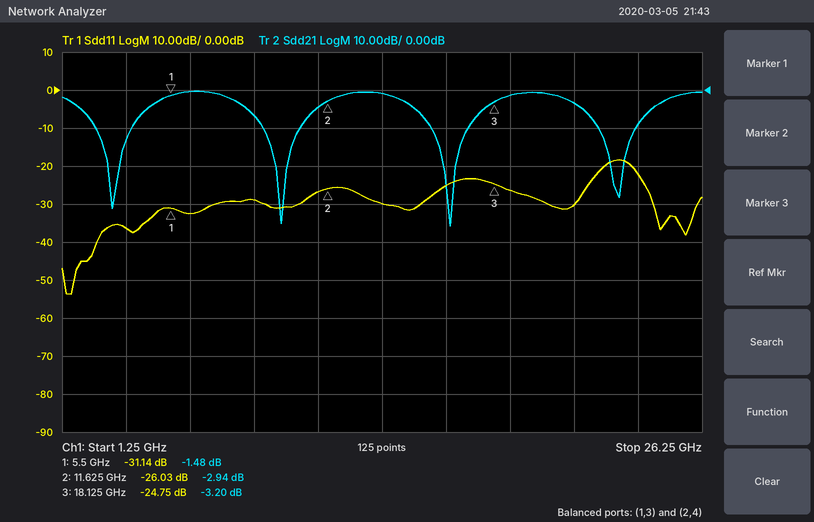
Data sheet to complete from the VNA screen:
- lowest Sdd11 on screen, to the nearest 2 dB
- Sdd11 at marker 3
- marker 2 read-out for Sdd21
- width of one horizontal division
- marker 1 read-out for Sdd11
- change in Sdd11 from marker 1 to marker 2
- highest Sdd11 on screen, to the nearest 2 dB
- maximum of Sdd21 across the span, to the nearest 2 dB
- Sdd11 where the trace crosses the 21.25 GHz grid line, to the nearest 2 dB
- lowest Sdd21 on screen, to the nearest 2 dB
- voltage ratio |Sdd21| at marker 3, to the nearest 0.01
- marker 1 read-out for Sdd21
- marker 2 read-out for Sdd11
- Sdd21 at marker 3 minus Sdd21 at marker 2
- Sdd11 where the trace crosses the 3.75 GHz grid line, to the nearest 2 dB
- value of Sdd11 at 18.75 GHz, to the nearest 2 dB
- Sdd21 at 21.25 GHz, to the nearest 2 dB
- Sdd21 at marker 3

-54 dB
-24.75 dB
-2.94 dB
2.5 GHz
-31.14 dB
5.11 dB
-18 dB
0 dB
-30 dB
-36 dB
0.69
-1.48 dB
-26.03 dB
-0.26 dB
-36 dB
-26 dB
-4 dB
-3.20 dB
